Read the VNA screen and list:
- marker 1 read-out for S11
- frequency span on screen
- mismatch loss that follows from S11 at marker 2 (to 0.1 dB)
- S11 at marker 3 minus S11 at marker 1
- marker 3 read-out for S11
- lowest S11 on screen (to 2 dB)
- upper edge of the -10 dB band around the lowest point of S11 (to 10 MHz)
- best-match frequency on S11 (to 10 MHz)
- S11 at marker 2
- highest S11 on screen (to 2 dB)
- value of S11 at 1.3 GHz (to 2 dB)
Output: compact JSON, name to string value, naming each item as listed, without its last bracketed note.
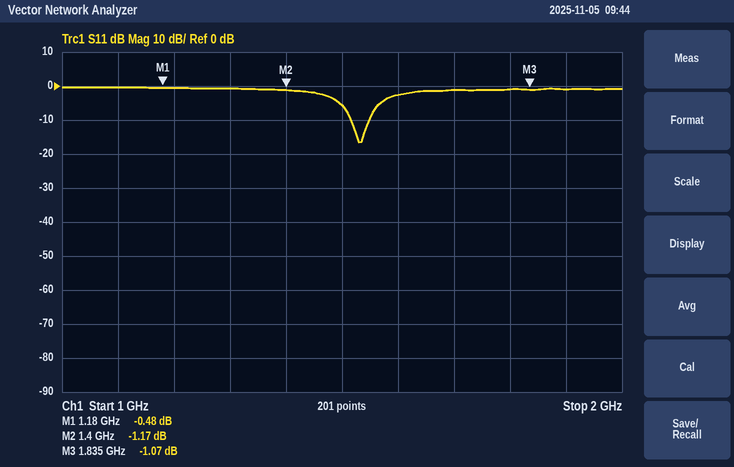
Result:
{"marker 1 read-out for S11": "-0.48 dB", "frequency span on screen": "1 GHz", "mismatch loss that follows from S11 at marker 2": "6.3 dB", "S11 at marker 3 minus S11 at marker 1": "-0.59 dB", "marker 3 read-out for S11": "-1.07 dB", "lowest S11 on screen": "-16 dB", "upper edge of the -10 dB band around the lowest point of S11": "1.55 GHz", "best-match frequency on S11": "1.53 GHz", "S11 at marker 2": "-1.17 dB", "highest S11 on screen": "0 dB", "value of S11 at 1.3 GHz": "0 dB"}
